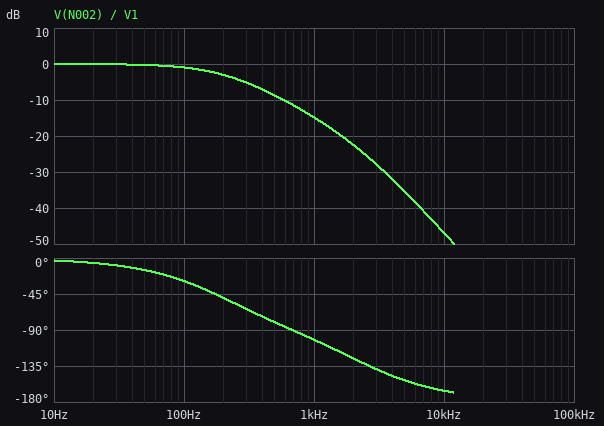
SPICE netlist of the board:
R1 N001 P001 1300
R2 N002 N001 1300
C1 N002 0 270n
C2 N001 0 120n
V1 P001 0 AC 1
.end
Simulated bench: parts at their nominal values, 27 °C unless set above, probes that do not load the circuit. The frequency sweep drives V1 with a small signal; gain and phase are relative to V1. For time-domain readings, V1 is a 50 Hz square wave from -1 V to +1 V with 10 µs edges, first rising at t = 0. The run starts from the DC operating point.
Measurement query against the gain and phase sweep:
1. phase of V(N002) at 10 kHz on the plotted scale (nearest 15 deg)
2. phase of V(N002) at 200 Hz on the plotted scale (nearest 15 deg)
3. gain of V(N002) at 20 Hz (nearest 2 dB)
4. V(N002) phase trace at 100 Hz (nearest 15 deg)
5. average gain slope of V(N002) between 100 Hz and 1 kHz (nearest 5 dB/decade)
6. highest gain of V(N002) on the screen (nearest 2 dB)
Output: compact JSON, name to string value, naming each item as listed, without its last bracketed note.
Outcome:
{"phase of V(N002) at 10 kHz on the plotted scale": "-165 deg", "phase of V(N002) at 200 Hz on the plotted scale": "-45 deg", "gain of V(N002) at 20 Hz": "0 dB", "V(N002) phase trace at 100 Hz": "-30 deg", "average gain slope of V(N002) between 100 Hz and 1 kHz": "-15 dB/decade", "highest gain of V(N002) on the screen": "0 dB"}
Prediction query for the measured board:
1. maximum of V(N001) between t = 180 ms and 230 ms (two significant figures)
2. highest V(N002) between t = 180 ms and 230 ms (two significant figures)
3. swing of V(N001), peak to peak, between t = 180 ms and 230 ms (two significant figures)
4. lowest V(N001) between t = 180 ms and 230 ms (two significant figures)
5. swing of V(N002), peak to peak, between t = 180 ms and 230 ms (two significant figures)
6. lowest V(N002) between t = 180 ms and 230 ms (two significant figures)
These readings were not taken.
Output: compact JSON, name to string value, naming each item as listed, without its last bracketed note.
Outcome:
{"maximum of V(N001) between t = 180 ms and 230 ms": "1.0 V", "highest V(N002) between t = 180 ms and 230 ms": "1.0 V", "swing of V(N001), peak to peak, between t = 180 ms and 230 ms": "2.0 V", "lowest V(N001) between t = 180 ms and 230 ms": "-1.0 V", "swing of V(N002), peak to peak, between t = 180 ms and 230 ms": "2.0 V", "lowest V(N002) between t = 180 ms and 230 ms": "-1.0 V"}
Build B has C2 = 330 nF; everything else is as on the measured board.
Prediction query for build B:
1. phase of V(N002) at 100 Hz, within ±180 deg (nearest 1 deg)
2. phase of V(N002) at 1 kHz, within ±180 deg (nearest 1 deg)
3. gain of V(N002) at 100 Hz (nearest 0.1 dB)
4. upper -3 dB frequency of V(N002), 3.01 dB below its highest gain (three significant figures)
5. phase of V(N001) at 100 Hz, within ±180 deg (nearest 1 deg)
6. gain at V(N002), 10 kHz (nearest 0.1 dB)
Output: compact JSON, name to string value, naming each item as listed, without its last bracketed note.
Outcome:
{"phase of V(N002) at 100 Hz, within ±180 deg": "-37 deg", "phase of V(N002) at 1 kHz, within ±180 deg": "-125 deg", "gain of V(N002) at 100 Hz": "-1.4 dB", "upper -3 dB frequency of V(N002), 3.01 dB below its highest gain": "159 Hz", "phase of V(N001) at 100 Hz, within ±180 deg": "-25 deg", "gain at V(N002), 10 kHz": "-55.5 dB"}
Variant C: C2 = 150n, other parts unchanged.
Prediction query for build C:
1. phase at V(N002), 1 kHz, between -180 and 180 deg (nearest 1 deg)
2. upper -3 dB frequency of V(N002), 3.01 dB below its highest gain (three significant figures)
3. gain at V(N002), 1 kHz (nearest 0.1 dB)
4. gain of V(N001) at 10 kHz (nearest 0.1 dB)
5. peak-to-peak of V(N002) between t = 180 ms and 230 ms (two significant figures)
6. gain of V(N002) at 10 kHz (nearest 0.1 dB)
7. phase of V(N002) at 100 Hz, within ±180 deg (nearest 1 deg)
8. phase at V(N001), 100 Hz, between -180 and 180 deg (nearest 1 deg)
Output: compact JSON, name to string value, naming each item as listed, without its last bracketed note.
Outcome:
{"phase at V(N002), 1 kHz, between -180 and 180 deg": "-107 deg", "upper -3 dB frequency of V(N002), 3.01 dB below its highest gain": "194 Hz", "gain at V(N002), 1 kHz": "-15.4 dB", "gain of V(N001) at 10 kHz": "-21.9 dB", "peak-to-peak of V(N002) between t = 180 ms and 230 ms": "2.0 V", "gain of V(N002) at 10 kHz": "-48.8 dB", "phase of V(N002) at 100 Hz, within ±180 deg": "-30 deg", "phase at V(N001), 100 Hz, between -180 and 180 deg": "-18 deg"}
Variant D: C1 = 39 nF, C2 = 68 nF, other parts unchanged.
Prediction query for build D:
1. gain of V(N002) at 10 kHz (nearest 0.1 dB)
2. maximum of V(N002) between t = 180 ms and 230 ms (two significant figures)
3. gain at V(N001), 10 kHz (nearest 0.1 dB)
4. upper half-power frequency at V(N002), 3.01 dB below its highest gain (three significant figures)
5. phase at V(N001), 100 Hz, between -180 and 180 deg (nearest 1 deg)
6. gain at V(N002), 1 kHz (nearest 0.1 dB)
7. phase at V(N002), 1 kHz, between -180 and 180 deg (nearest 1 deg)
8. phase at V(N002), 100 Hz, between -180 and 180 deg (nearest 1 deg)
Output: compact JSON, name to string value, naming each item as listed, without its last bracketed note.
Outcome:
{"gain of V(N002) at 10 kHz": "-26.2 dB", "maximum of V(N002) between t = 180 ms and 230 ms": "1.0 V", "gain at V(N001), 10 kHz": "-15.8 dB", "upper half-power frequency at V(N002), 3.01 dB below its highest gain": "955 Hz", "phase at V(N001), 100 Hz, between -180 and 180 deg": "-5 deg", "gain at V(N002), 1 kHz": "-3.2 dB", "phase at V(N002), 1 kHz, between -180 and 180 deg": "-55 deg", "phase at V(N002), 100 Hz, between -180 and 180 deg": "-7 deg"}
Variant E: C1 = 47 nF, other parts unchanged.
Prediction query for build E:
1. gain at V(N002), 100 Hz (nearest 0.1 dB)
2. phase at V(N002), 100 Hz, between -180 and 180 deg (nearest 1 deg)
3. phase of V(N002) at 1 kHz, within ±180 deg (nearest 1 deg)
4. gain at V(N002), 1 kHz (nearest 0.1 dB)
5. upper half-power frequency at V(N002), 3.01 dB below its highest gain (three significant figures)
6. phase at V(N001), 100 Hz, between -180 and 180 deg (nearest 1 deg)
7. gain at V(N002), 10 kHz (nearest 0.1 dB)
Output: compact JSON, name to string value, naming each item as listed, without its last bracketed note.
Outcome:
{"gain at V(N002), 100 Hz": "-0.1 dB", "phase at V(N002), 100 Hz, between -180 and 180 deg": "-10 deg", "phase of V(N002) at 1 kHz, within ±180 deg": "-70 deg", "gain at V(N002), 1 kHz": "-5.4 dB", "upper half-power frequency at V(N002), 3.01 dB below its highest gain": "651 Hz", "phase at V(N001), 100 Hz, between -180 and 180 deg": "-8 deg", "gain at V(N002), 10 kHz": "-32.2 dB"}
